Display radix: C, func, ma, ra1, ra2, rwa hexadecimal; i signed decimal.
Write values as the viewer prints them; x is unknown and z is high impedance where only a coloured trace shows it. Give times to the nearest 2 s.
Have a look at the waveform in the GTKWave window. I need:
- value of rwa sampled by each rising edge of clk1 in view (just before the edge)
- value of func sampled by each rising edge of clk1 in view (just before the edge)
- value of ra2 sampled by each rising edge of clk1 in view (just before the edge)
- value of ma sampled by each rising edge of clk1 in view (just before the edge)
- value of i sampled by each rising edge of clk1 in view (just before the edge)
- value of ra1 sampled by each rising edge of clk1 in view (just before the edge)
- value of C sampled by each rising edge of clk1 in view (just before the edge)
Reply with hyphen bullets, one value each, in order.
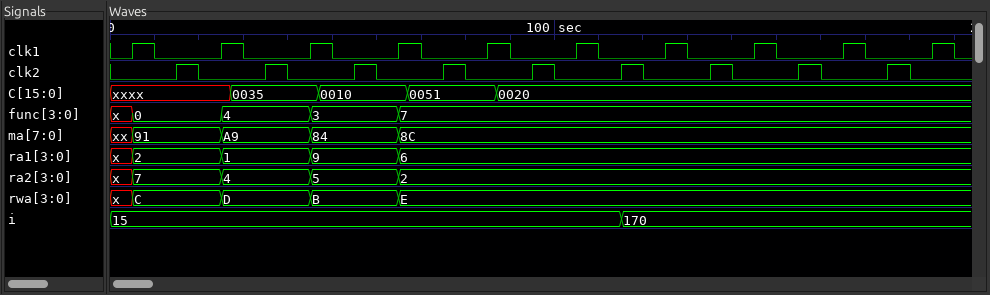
- x, C, D, B, E, E, E, E, E, E
- x, 0, 4, 3, 7, 7, 7, 7, 7, 7
- x, 7, 4, 5, 2, 2, 2, 2, 2, 2
- xx, 91, A9, 84, 8C, 8C, 8C, 8C, 8C, 8C
- 15, 15, 15, 15, 15, 15, 170, 170, 170, 170
- x, 2, 1, 9, 6, 6, 6, 6, 6, 6
- xxxx, xxxx, 0035, 0010, 0051, 0020, 0020, 0020, 0020, 0020
